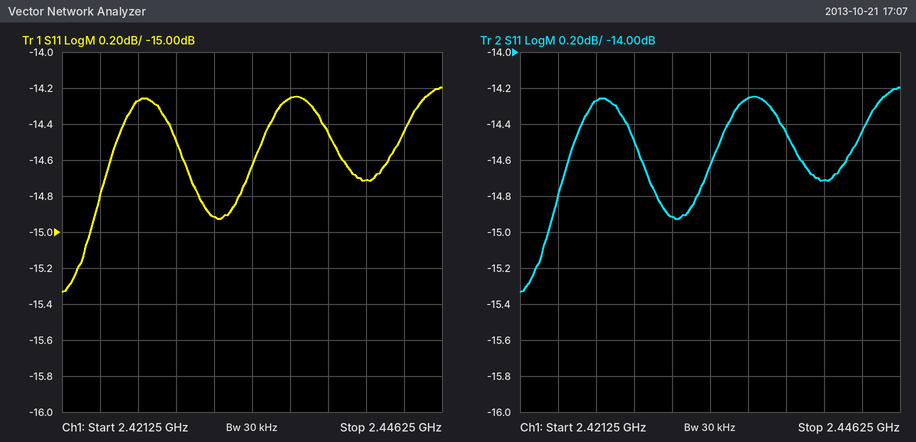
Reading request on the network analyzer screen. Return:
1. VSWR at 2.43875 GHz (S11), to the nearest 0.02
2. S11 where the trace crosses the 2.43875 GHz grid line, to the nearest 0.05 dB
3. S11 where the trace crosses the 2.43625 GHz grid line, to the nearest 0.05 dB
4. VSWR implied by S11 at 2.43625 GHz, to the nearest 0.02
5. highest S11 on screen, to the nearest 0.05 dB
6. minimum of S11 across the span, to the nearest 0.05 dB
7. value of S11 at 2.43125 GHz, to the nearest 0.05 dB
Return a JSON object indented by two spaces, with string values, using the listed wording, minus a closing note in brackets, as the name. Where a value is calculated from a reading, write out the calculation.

{
  "VSWR at 2.43875 GHz (S11), to the nearest 0.02": "|Γ| = 10^(-14.45/20) = 0.1895; VSWR = (1 + 0.1895)/(1 − 0.1895) ≈ 1.47, so 1.46 to the nearest 0.02",
  "S11 where the trace crosses the 2.43875 GHz grid line, to the nearest 0.05 dB": "-14.45 dB",
  "S11 where the trace crosses the 2.43625 GHz grid line, to the nearest 0.05 dB": "-14.25 dB",
  "VSWR implied by S11 at 2.43625 GHz, to the nearest 0.02": "|Γ| = 10^(-14.25/20) = 0.1939; VSWR = (1 + 0.1939)/(1 − 0.1939) ≈ 1.48",
  "highest S11 on screen, to the nearest 0.05 dB": "-14.20 dB",
  "minimum of S11 across the span, to the nearest 0.05 dB": "-15.35 dB",
  "value of S11 at 2.43125 GHz, to the nearest 0.05 dB": "-14.90 dB"
}
